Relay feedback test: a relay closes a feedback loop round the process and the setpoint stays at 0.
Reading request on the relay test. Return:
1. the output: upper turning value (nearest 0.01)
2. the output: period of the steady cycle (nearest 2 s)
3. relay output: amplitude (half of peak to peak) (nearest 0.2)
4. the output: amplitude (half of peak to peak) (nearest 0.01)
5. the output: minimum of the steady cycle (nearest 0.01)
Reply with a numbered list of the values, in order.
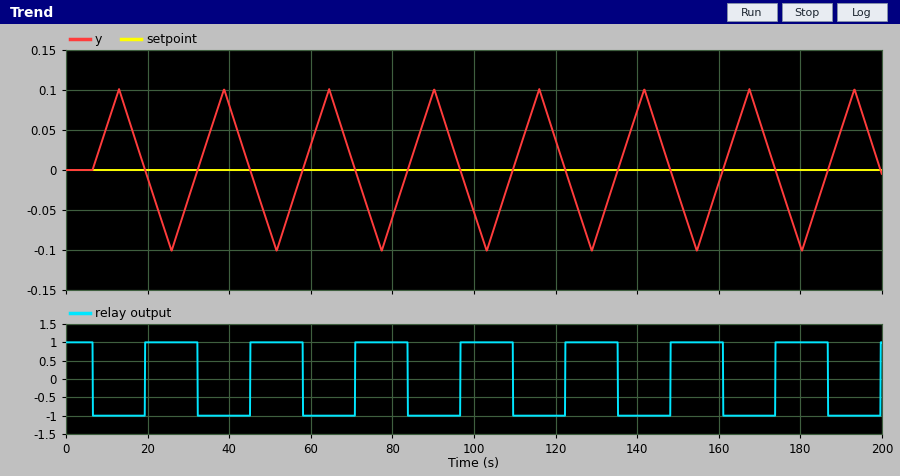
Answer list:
1. 0.10
2. 26 s
3. 1.0
4. 0.10
5. -0.10
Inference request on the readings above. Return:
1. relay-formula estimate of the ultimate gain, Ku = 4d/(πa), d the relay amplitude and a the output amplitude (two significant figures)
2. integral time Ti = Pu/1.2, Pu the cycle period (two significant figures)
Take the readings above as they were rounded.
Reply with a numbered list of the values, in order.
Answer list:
1. 13
2. 22 s
